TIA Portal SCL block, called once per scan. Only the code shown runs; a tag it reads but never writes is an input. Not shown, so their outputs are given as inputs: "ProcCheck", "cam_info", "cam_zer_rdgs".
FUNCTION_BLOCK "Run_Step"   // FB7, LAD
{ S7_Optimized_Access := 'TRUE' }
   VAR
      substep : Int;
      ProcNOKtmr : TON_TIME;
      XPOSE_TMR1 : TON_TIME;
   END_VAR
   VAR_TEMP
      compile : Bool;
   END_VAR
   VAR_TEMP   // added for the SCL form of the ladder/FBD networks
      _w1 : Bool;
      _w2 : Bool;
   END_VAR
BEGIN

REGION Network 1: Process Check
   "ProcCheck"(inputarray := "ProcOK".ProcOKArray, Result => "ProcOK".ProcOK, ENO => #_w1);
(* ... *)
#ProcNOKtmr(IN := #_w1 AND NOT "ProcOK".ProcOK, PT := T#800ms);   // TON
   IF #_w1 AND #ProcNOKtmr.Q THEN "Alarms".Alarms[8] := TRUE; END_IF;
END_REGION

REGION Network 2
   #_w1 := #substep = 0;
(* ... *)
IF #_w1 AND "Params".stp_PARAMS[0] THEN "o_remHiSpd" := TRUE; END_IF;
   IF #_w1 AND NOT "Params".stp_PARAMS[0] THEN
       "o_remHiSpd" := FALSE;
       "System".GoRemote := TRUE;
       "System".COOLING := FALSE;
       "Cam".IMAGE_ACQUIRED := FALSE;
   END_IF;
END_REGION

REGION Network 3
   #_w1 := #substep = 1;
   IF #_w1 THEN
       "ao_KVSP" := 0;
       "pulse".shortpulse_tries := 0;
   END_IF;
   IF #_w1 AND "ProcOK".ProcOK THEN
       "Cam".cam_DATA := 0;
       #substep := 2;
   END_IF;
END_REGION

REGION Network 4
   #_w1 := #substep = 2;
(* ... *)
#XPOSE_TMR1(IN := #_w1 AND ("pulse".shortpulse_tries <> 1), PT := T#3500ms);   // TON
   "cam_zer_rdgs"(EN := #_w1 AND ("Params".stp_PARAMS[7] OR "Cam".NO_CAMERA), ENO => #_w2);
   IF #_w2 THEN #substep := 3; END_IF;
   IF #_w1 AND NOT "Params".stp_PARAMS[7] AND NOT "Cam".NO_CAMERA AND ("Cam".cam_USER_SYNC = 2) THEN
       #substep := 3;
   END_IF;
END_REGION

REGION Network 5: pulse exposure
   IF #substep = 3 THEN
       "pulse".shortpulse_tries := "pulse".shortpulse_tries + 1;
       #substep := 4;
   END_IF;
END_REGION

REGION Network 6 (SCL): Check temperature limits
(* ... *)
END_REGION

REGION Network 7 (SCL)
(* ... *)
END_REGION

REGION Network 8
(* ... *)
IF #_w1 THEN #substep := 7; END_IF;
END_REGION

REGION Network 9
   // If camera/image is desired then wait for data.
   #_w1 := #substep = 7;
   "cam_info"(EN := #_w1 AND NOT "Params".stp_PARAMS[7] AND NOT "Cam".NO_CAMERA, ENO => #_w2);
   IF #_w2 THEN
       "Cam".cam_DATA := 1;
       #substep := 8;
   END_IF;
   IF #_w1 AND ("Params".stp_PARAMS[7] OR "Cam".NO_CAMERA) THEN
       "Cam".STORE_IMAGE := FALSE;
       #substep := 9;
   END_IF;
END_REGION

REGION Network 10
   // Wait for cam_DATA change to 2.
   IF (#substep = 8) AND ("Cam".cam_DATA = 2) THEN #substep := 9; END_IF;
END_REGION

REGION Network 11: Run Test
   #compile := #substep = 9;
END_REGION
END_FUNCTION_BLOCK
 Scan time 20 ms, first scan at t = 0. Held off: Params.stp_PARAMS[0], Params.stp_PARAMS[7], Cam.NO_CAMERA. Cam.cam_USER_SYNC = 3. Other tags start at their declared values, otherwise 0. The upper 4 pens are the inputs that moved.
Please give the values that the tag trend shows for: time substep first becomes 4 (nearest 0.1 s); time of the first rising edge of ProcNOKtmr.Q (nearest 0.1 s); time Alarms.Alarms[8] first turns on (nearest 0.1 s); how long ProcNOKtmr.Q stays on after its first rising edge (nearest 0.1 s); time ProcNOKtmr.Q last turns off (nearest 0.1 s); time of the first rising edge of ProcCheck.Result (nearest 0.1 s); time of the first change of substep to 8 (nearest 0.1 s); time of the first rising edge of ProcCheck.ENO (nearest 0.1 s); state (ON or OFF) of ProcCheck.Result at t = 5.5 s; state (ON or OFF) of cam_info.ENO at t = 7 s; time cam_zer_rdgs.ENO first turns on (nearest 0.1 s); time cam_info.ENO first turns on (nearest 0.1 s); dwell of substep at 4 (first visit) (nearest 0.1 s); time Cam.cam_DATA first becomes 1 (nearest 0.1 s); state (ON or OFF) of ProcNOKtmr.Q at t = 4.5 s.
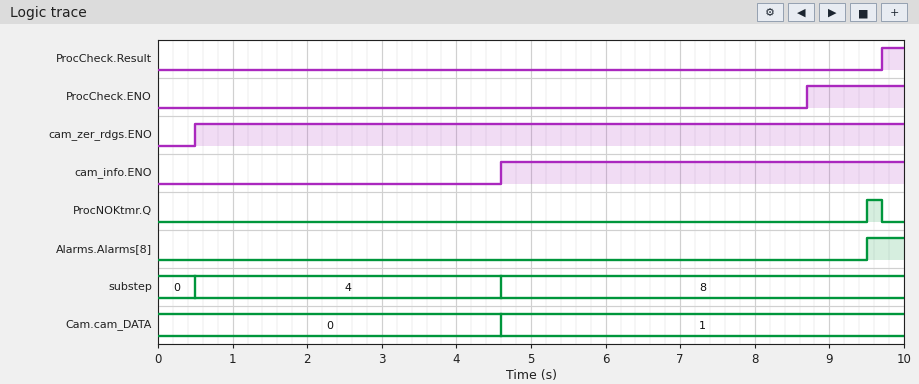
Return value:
0.5 s
9.5 s
9.5 s
0.2 s
9.7 s
9.7 s
4.6 s
8.7 s
OFF
ON
0.5 s
4.6 s
4.1 s
4.6 s
OFF
